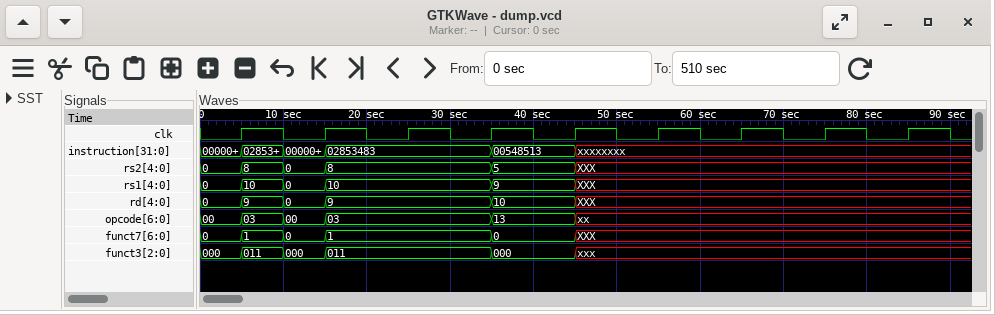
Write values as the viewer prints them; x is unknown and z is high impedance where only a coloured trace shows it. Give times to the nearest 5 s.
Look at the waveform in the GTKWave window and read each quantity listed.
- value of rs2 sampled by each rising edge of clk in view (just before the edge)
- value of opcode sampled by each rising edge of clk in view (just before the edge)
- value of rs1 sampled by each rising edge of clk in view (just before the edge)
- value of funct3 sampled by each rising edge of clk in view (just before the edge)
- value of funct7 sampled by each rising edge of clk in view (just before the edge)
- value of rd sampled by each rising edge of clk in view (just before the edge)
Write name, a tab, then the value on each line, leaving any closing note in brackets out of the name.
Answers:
value of rs2 sampled by each rising edge of clk in view	0, 0, 8, 8, 5, XXX, XXX, XXX, XXX
value of opcode sampled by each rising edge of clk in view	00, 00, 03, 03, 13, xx, xx, xx, xx
value of rs1 sampled by each rising edge of clk in view	0, 0, 10, 10, 9, XXX, XXX, XXX, XXX
value of funct3 sampled by each rising edge of clk in view	000, 000, 011, 011, 000, xxx, xxx, xxx, xxx
value of funct7 sampled by each rising edge of clk in view	0, 0, 1, 1, 0, XXX, XXX, XXX, XXX
value of rd sampled by each rising edge of clk in view	0, 0, 9, 9, 10, XXX, XXX, XXX, XXX
